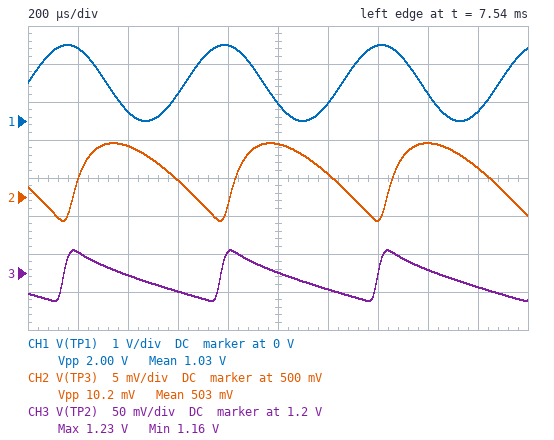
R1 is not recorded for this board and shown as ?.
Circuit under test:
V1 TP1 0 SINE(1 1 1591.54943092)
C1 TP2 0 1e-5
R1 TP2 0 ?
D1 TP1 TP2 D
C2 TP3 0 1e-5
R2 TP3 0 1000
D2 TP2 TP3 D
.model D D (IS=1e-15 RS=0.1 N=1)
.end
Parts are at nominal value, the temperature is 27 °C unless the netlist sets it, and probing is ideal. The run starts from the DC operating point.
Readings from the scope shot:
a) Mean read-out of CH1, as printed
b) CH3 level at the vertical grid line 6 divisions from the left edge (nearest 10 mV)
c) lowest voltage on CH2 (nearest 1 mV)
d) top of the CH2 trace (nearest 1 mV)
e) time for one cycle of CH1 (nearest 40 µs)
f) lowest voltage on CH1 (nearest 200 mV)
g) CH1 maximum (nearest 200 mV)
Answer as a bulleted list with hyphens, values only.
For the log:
- 1.03 V
- 1.18 V
- 497 mV
- 507 mV
- 640 µs
- 0 V
- 2.0 V
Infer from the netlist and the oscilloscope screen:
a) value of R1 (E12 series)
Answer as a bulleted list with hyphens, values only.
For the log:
- 1.5 kΩ
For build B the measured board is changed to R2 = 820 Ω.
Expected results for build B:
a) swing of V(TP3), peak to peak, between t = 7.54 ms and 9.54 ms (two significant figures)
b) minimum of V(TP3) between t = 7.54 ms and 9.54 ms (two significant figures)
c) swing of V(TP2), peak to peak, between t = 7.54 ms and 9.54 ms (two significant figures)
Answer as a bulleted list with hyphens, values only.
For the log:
- 13 mV
- 490 mV
- 70 mV
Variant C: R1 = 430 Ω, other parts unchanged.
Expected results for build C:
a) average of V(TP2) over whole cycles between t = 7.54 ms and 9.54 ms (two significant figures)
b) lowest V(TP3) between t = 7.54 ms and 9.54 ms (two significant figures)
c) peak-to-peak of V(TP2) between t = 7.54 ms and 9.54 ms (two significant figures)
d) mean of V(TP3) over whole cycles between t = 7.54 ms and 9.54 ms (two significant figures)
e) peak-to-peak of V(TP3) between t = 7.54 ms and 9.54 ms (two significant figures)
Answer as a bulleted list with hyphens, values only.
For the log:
- 1.1 V
- 470 mV
- 160 mV
- 480 mV
- 18 mV
